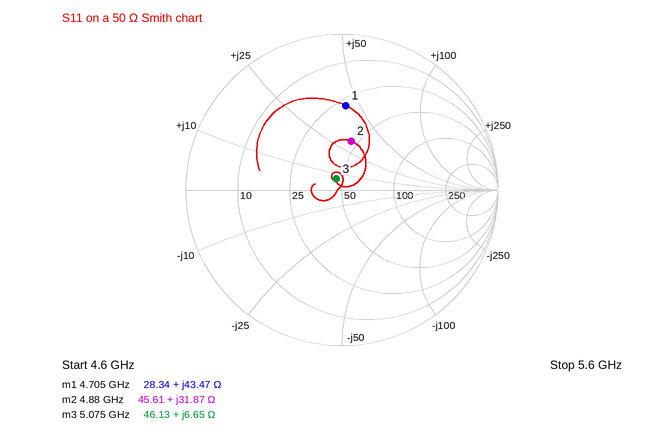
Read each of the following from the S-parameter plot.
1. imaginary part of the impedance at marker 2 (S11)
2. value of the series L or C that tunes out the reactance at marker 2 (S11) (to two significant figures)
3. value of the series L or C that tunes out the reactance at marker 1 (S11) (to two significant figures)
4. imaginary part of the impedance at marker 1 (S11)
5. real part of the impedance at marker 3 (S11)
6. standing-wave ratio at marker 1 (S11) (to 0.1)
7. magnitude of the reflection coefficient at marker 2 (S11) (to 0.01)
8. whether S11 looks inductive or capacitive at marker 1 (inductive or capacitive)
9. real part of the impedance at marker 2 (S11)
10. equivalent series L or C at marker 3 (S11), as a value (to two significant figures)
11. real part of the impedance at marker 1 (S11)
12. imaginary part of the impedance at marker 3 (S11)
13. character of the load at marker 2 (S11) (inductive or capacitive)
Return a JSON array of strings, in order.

["+31.87 Ω", "1.0 pF", "780 fF", "+43.47 Ω", "46.13 Ω", "3.4", "0.32", "inductive", "45.61 Ω", "210 pH", "28.34 Ω", "+6.65 Ω", "inductive"]
